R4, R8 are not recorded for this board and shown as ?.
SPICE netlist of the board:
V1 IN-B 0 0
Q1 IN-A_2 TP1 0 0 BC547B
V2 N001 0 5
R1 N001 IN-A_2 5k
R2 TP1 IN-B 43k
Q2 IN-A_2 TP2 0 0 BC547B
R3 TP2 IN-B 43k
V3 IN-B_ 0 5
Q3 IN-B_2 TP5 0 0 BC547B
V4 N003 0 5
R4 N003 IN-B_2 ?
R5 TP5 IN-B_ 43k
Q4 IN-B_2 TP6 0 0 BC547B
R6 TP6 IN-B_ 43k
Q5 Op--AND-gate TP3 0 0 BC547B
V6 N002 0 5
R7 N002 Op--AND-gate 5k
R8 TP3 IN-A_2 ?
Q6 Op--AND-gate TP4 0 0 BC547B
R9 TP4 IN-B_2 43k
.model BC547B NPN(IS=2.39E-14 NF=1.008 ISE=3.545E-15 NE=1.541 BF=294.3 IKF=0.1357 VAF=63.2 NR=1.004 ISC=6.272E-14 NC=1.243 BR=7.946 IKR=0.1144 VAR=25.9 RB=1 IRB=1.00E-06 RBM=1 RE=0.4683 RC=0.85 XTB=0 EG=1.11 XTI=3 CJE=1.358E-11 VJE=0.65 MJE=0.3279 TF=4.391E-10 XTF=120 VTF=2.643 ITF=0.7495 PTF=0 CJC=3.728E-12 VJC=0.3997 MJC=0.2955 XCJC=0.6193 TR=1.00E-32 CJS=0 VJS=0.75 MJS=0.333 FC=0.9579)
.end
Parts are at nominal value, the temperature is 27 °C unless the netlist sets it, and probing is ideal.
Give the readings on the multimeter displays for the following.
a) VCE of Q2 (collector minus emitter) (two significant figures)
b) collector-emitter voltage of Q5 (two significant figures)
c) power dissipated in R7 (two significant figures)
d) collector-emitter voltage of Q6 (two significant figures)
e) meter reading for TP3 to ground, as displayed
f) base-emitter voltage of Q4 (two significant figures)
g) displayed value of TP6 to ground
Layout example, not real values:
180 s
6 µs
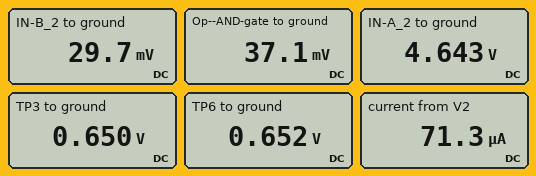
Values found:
4.6 V
37 mV
4.9 mW
37 mV
0.650 V
650 mV
0.652 V
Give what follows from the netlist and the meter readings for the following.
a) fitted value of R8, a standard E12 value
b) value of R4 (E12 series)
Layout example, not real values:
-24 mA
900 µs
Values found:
56 kΩ
2.7 kΩ
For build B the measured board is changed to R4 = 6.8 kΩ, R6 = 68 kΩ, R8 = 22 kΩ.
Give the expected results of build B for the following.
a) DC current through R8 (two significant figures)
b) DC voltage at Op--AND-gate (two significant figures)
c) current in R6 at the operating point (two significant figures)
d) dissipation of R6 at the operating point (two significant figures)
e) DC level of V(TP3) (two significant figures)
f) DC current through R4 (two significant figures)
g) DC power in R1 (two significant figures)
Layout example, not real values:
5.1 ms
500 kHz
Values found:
160 µA
24 mV
64 µA
280 µW
660 mV
730 µA
130 µW
